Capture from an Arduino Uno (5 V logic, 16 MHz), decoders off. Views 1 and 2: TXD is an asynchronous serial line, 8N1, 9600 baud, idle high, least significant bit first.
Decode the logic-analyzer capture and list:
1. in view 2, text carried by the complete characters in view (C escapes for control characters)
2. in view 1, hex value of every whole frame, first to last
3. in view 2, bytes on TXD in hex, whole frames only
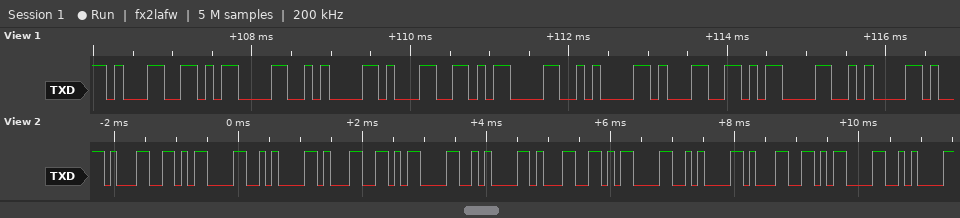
"1\r\n1\r\n1\r\n1\r\n"
0x31 0x0D 0x0A 0x31 0x0D 0x0A 0x31 0x0D 0x0A
31 0D 0A 31 0D 0A 31 0D 0A 31 0D 0A
